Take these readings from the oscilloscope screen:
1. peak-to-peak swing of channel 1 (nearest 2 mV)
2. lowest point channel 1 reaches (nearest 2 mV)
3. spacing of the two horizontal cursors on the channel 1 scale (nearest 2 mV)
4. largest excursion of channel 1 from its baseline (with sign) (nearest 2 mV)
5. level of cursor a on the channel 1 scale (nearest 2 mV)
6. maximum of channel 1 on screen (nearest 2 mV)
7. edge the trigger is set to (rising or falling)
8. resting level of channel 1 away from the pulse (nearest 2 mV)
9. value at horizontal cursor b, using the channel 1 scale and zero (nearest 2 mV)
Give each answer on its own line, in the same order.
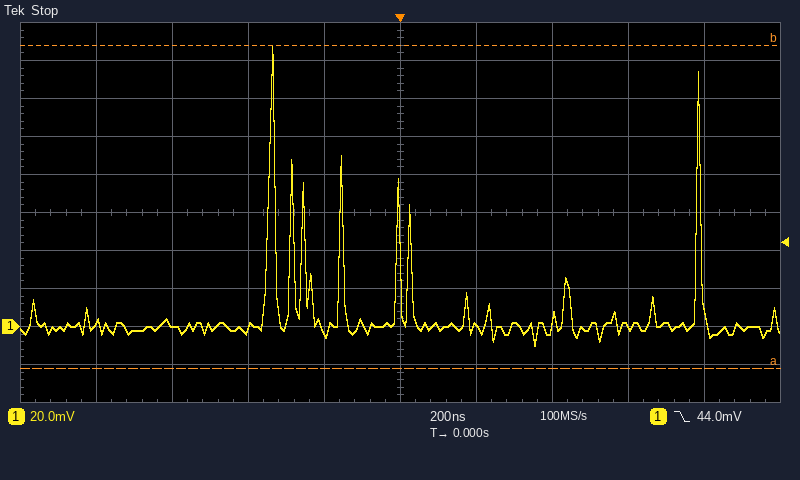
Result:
158 mV
-10 mV
170 mV
+148 mV
-22 mV
148 mV
falling
0 mV
148 mV
